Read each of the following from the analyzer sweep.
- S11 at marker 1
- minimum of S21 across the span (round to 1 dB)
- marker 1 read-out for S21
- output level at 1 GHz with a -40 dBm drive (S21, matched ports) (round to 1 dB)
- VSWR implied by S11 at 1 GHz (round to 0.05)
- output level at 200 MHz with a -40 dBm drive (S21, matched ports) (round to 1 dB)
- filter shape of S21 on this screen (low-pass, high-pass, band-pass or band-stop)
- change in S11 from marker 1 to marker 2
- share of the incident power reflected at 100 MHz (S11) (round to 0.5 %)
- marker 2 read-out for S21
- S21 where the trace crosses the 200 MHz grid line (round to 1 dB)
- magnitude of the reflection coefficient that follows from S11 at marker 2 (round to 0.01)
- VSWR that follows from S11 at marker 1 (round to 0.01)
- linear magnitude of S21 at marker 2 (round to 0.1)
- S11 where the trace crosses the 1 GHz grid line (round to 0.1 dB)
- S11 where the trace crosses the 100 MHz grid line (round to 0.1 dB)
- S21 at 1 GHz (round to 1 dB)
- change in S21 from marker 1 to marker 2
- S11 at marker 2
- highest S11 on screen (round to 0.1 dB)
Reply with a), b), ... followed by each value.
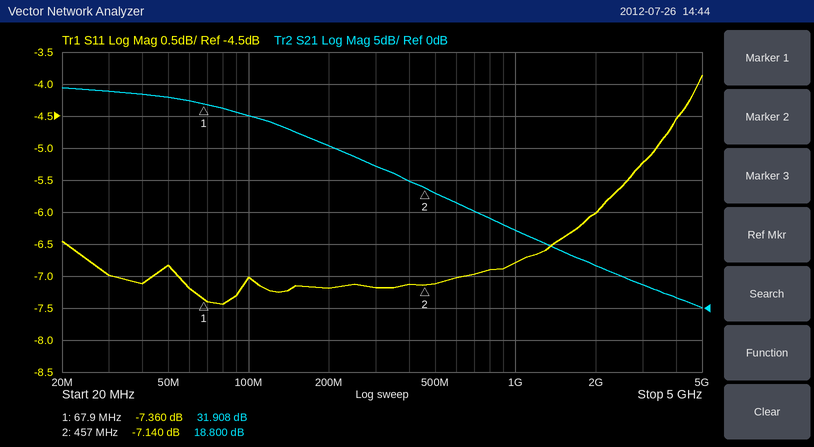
a) -7.360 dB
b) 0 dB
c) 31.908 dB
d) -28 dBm
e) 2.70
f) -15 dBm
g) low-pass
h) 0.220 dB
i) 20.0 %
j) 18.800 dB
k) 25 dB
l) 0.44
m) 2.50
n) 8.7
o) -6.8 dB
p) -7.0 dB
q) 12 dB
r) -13.108 dB
s) -7.140 dB
t) -3.9 dB
